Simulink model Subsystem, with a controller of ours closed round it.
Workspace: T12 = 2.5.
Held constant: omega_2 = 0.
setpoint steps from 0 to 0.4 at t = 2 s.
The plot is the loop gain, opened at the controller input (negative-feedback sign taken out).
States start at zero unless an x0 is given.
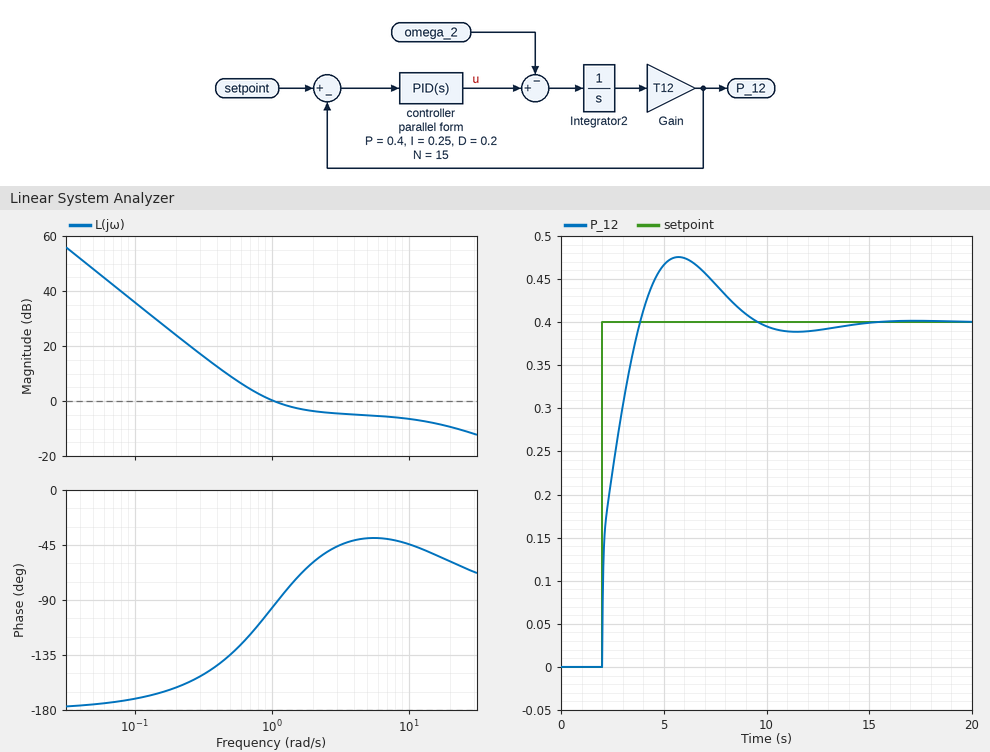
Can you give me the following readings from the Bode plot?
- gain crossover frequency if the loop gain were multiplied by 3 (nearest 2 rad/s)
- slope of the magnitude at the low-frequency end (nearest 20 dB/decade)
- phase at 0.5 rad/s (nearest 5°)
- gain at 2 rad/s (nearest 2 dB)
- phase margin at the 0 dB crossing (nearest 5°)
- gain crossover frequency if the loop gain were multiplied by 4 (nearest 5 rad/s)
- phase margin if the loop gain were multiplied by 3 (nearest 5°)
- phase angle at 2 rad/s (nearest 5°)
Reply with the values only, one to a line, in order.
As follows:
20 rad/s
-40 dB/decade
-135°
-4 dB
85°
30 rad/s
120°
-60°
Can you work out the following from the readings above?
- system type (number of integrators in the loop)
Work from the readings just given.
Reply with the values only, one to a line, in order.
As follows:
2
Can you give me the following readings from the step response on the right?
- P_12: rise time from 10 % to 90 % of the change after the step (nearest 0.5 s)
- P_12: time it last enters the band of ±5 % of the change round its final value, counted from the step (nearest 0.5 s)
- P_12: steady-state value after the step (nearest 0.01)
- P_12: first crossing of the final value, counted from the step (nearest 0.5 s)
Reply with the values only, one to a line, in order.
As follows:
1.5 s
6.5 s
0.40
2.0 s
